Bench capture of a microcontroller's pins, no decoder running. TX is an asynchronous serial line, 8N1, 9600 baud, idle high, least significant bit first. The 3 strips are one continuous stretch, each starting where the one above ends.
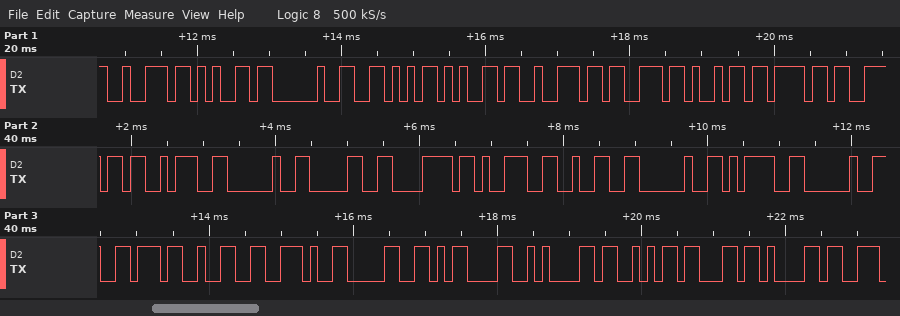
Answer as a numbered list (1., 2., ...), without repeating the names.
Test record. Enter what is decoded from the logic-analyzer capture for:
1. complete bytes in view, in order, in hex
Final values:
1. 0x72 0x65 0x20 0x56 0x65 0x72 0x73 0x69 0x6F 0x6E 0x3A 0x20 0x30 0x78 0x39 0x32 0x20 0x3D 0x20 0x76 0x32 0x2E 0x30 0x0D 0x0A 0x53 0x63 0x61
